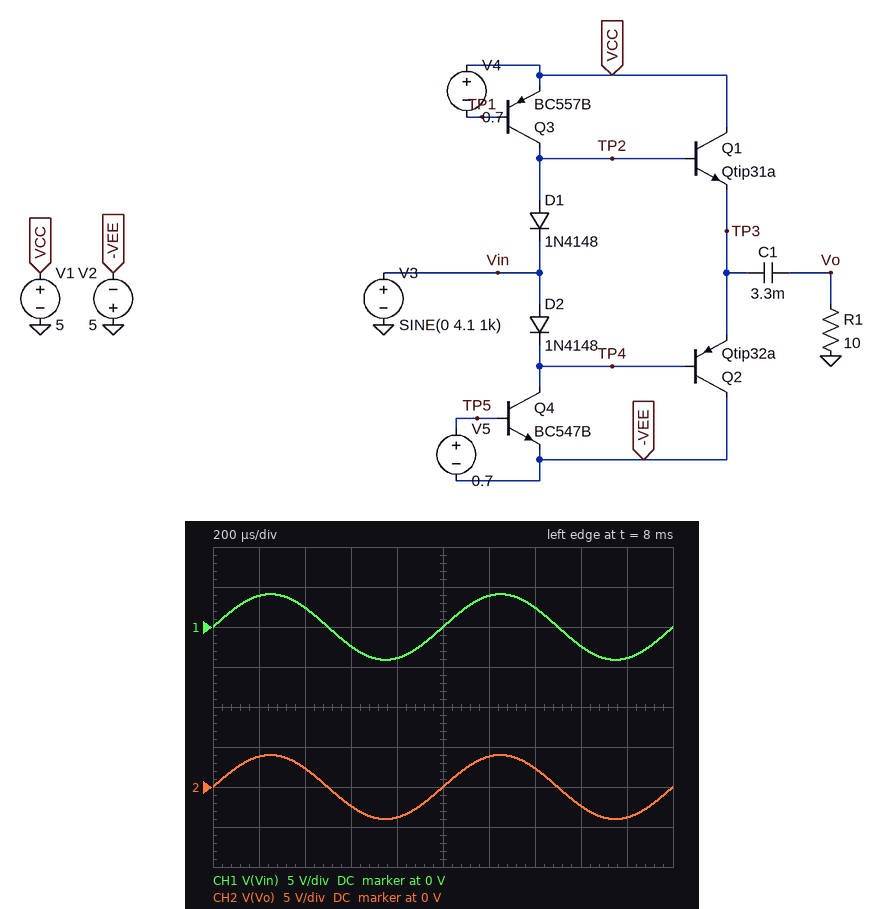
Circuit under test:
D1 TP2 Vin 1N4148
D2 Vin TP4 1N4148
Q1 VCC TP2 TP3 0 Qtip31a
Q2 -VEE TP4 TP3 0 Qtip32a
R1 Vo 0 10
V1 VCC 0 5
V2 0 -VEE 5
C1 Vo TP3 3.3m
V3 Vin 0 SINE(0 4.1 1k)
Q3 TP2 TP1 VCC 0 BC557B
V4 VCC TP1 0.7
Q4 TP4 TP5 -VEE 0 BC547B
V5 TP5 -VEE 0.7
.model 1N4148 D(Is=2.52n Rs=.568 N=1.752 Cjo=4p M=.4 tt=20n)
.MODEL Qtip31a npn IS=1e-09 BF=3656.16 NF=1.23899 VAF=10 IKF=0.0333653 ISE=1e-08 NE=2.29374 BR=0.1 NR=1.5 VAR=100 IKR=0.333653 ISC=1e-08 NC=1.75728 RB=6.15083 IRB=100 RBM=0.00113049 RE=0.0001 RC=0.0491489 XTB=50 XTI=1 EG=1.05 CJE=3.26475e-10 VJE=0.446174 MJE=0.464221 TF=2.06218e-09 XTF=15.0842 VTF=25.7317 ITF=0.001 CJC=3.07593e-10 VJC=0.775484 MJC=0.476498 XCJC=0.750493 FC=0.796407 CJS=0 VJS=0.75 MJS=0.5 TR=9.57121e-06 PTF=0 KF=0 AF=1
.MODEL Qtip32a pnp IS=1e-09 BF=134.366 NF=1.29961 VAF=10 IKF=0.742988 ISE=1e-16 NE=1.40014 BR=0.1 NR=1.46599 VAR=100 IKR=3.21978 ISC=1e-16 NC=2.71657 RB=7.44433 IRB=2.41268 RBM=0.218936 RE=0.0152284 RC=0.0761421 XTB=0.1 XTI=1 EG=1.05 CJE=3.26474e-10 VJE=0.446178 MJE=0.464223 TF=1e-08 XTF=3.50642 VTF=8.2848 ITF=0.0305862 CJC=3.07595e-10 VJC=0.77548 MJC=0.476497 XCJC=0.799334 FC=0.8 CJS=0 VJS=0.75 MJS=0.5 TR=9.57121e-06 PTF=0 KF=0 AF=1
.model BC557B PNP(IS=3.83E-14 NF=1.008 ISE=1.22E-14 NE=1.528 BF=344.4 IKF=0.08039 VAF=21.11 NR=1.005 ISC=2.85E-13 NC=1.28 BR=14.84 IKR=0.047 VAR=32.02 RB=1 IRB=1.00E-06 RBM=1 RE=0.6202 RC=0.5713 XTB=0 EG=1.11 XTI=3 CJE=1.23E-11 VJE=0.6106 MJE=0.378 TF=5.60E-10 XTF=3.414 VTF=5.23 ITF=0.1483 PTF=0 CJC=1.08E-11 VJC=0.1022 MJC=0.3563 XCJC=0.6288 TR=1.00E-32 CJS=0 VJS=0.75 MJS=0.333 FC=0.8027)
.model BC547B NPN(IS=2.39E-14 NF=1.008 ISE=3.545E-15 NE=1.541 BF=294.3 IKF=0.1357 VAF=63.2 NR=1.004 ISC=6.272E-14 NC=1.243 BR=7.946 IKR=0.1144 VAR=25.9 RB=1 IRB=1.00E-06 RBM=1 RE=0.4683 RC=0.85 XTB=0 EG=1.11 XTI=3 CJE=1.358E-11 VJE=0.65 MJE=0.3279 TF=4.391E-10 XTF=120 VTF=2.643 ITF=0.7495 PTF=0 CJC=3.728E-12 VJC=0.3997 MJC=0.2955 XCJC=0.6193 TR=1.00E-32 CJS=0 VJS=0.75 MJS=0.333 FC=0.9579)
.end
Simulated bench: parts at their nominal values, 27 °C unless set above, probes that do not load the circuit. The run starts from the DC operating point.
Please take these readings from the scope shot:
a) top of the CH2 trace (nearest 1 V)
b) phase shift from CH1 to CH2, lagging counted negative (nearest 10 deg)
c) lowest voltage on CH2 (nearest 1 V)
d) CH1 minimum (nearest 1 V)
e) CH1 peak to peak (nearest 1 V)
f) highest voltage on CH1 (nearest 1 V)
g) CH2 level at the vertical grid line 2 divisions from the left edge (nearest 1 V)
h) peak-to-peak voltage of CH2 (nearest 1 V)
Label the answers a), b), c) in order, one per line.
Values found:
a) 4 V
b) 0 deg
c) -4 V
d) -4 V
e) 8 V
f) 4 V
g) 2 V
h) 8 V
